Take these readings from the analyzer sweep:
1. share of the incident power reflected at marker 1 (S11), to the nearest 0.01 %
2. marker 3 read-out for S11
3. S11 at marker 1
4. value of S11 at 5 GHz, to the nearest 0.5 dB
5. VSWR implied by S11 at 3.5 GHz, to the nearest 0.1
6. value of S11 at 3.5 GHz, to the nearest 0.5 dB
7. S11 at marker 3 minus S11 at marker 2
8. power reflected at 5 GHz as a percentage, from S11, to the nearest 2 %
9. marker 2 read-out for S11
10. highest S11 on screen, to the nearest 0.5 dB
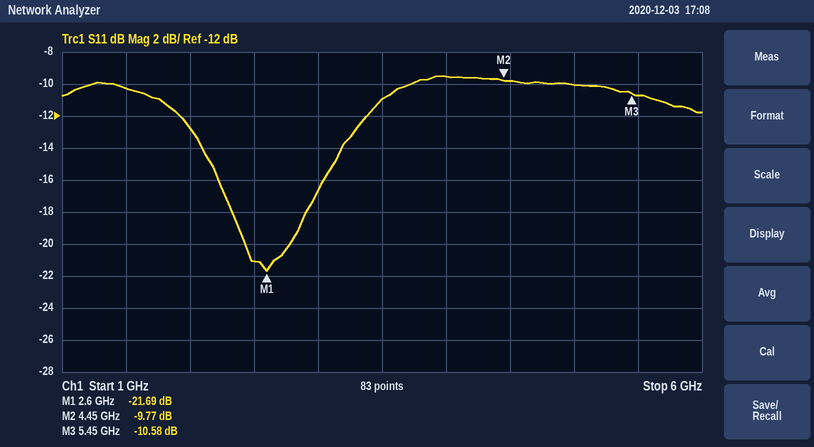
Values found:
0.68 %
-10.58 dB
-21.69 dB
-10.0 dB
1.8
-11.0 dB
-0.81 dB
10 %
-9.77 dB
-9.5 dB
